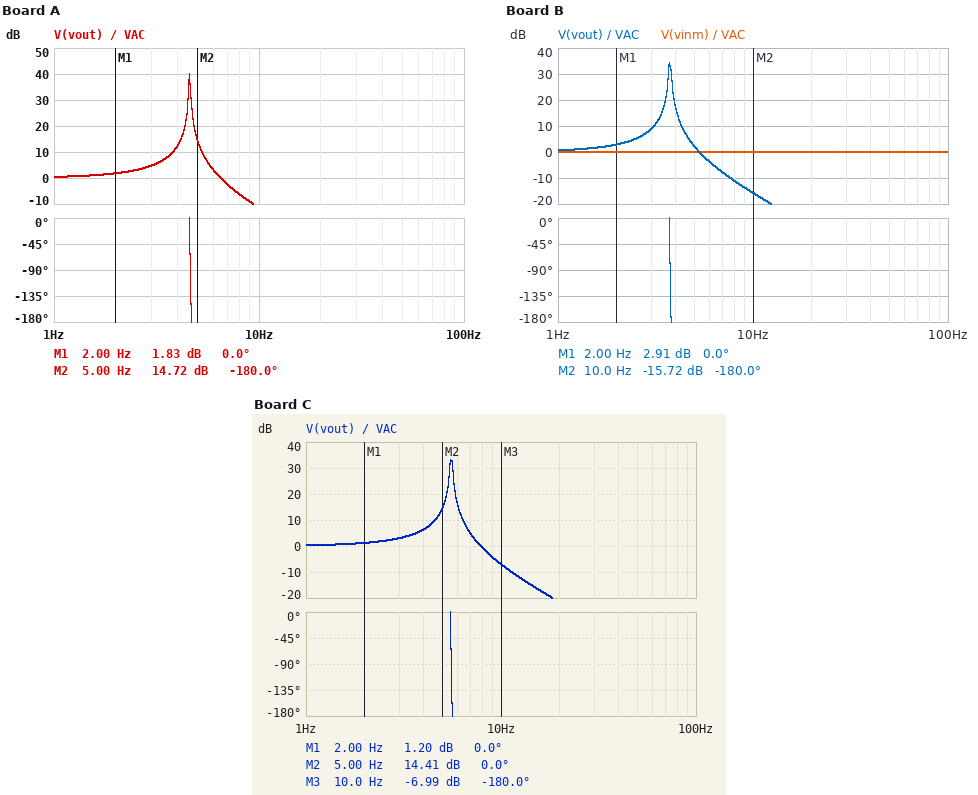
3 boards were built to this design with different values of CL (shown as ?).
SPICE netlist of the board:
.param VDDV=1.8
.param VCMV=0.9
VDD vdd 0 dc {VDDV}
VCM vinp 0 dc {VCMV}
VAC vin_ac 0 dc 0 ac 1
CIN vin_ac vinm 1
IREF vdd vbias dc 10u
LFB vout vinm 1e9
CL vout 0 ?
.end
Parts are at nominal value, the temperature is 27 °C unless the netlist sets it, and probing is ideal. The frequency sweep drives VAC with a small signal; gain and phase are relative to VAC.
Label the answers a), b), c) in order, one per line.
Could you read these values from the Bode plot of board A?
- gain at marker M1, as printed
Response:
a) 1.83 dB
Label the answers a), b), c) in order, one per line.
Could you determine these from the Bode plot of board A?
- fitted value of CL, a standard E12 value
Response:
a) 1.2 pF
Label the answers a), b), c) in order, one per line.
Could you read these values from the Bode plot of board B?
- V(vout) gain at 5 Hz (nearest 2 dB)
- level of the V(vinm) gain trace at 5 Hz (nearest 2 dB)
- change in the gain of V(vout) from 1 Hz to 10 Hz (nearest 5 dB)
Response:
a) 2 dB
b) 0 dB
c) -15 dB
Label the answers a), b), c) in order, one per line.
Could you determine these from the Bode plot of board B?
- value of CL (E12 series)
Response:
a) 1.8 pF
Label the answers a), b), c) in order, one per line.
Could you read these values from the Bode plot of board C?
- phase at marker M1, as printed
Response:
a) 0.0 deg
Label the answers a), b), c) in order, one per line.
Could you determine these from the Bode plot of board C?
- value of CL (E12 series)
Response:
a) 820 fF
